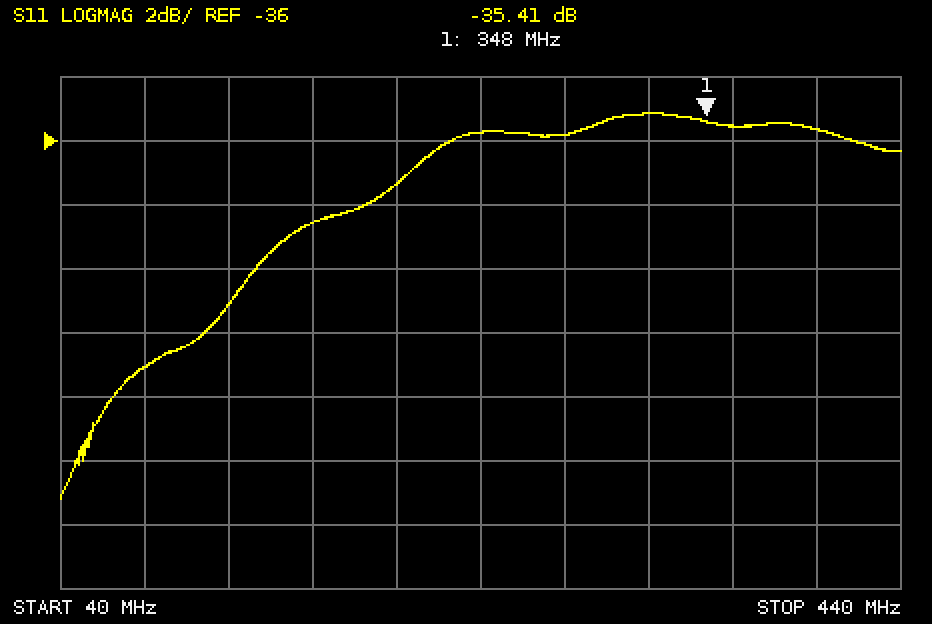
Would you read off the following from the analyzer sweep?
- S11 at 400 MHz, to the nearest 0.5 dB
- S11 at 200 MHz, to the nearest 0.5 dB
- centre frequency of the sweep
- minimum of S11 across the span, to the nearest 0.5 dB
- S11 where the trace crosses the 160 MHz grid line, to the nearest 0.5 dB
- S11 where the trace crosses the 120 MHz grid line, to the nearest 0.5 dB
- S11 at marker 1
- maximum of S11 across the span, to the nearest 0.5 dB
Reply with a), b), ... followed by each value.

a) -35.5 dB
b) -37.5 dB
c) 240 MHz
d) -47.0 dB
e) -38.5 dB
f) -41.0 dB
g) -35.41 dB
h) -35.0 dB
